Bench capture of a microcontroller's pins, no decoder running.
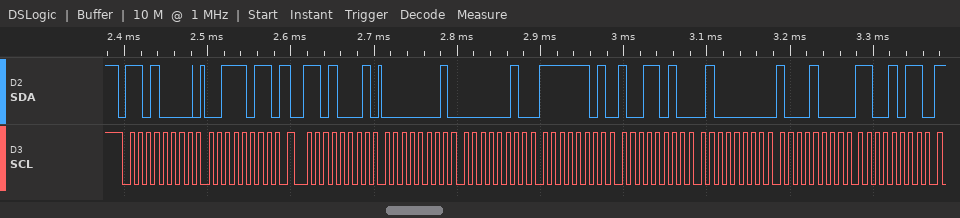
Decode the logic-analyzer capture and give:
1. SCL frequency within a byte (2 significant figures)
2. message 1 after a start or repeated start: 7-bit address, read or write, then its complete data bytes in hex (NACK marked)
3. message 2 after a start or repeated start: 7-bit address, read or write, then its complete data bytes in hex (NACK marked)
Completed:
100 kHz
0x68 write: 3B
0x68 read: 01 02 FD 9A 40 88 CB
